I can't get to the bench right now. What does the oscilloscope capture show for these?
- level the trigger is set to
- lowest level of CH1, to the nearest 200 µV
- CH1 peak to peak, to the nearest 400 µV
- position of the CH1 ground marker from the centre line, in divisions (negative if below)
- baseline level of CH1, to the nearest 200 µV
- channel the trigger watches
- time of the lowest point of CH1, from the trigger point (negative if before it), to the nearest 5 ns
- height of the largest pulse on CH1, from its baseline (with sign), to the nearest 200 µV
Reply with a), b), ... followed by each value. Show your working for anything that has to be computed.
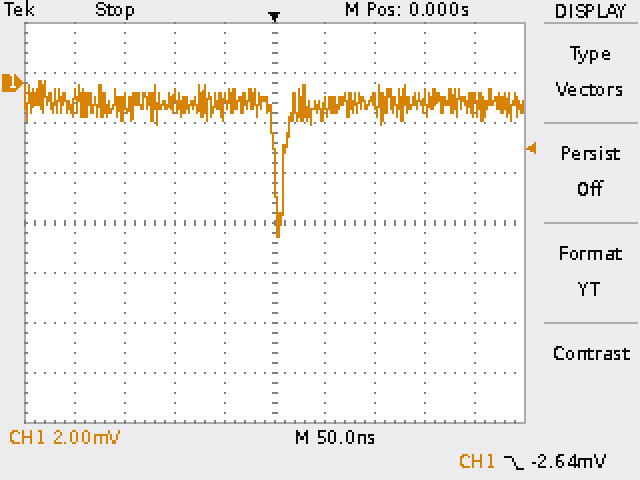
a) -2.64 mV
b) -6.2 mV
c) 6.4 mV
d) +2.8 div
e) -800 µV
f) CH1
g) +5 ns
h) -6.2 mV − (-800 µV) = -5.4 mV
